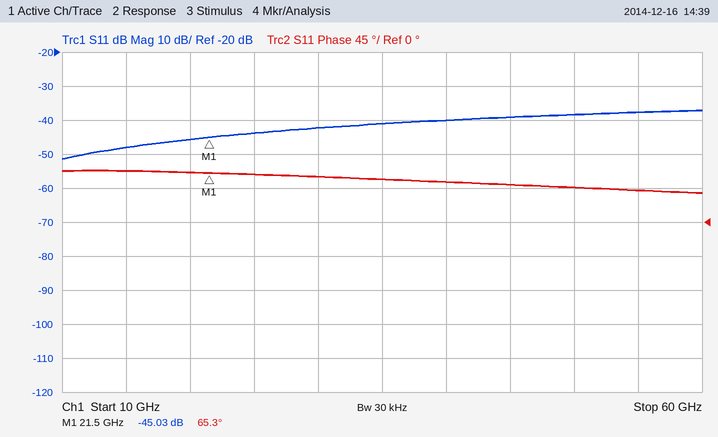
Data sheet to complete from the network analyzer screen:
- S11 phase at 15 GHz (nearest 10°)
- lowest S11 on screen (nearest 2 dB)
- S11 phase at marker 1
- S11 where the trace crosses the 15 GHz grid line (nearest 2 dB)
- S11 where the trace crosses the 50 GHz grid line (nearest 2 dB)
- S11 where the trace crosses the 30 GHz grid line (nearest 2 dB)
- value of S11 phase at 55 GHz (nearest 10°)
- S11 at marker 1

70°
-52 dB
65.3°
-48 dB
-38 dB
-42 dB
40°
-45.03 dB
